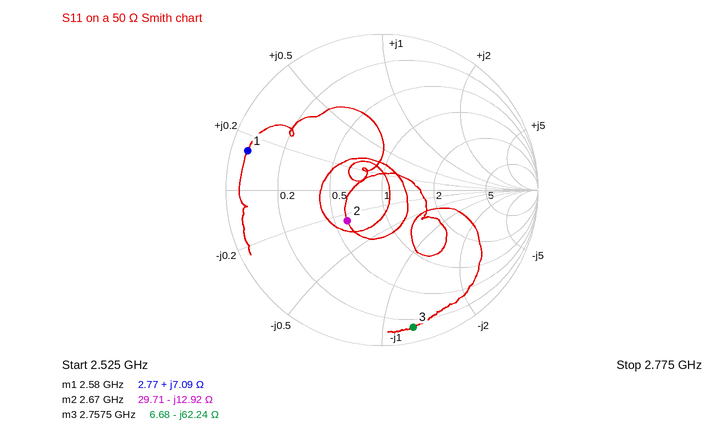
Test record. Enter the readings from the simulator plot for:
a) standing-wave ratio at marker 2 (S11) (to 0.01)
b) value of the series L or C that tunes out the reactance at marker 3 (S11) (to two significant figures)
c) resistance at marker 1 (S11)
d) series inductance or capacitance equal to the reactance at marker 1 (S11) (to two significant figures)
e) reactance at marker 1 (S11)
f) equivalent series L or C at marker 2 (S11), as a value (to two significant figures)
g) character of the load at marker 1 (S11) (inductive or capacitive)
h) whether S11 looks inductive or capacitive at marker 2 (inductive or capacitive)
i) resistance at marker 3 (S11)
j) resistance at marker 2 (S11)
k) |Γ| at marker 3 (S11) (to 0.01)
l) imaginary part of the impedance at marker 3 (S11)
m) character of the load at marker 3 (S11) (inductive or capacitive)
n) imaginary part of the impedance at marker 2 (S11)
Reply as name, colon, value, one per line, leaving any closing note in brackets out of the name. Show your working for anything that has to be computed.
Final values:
standing-wave ratio at marker 2 (S11): 1.85
value of the series L or C that tunes out the reactance at marker 3 (S11): L = 62.24 Ω/(2π × 2.7575 GHz) ≈ 3.6 nH
resistance at marker 1: 2.77 Ω
series inductance or capacitance equal to the reactance at marker 1 (S11): L = 7.09 Ω/(2π × 2.58 GHz) ≈ 437 pH, so 440 pH to two significant figures
reactance at marker 1: +7.09 Ω
equivalent series L or C at marker 2 (S11), as a value: C = 1/(2π × 2.67 GHz × 12.92 Ω) ≈ 4.6 pF
character of the load at marker 1 (S11): inductive
whether S11 looks inductive or capacitive at marker 2: capacitive
resistance at marker 3: 6.68 Ω
resistance at marker 2: 29.71 Ω
|Γ| at marker 3 (S11): 0.90
imaginary part of the impedance at marker 3: -62.24 Ω
character of the load at marker 3 (S11): capacitive
imaginary part of the impedance at marker 2: -12.92 Ω
